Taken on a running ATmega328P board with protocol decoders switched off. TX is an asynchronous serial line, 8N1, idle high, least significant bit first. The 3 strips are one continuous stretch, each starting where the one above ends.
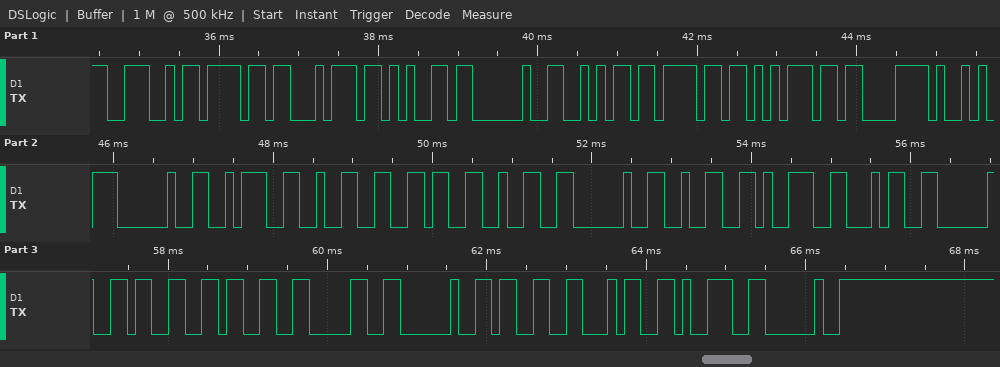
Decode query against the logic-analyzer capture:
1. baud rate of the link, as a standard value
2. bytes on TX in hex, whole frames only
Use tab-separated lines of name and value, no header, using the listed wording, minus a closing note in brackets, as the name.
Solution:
baud rate of the link, as a standard value	9600 baud
bytes on TX in hex, whole frames only	0x4E 0x6F 0x74 0x65 0x20 0x6A 0x6F 0x75 0xC3 0xA9 0x20 0x3A 0x32 0x36 0x32 0x20 0x32 0x39 0x34 0x20 0x33 0x33 0x30 0x20 0x33 0x34 0x39 0x20
